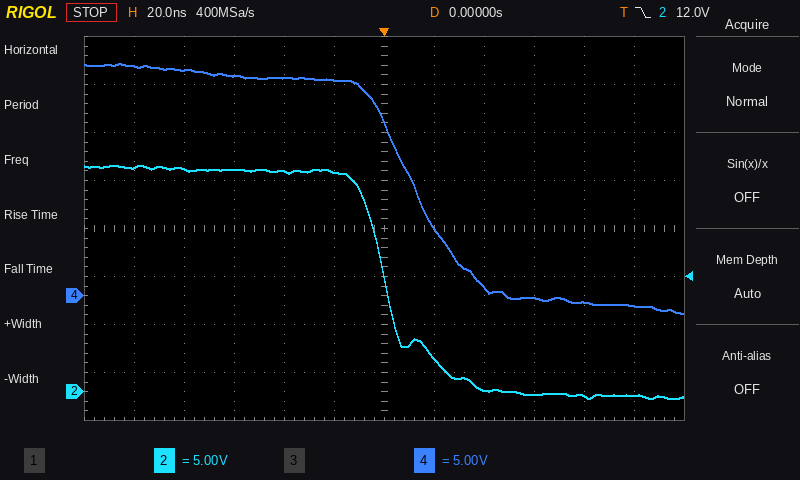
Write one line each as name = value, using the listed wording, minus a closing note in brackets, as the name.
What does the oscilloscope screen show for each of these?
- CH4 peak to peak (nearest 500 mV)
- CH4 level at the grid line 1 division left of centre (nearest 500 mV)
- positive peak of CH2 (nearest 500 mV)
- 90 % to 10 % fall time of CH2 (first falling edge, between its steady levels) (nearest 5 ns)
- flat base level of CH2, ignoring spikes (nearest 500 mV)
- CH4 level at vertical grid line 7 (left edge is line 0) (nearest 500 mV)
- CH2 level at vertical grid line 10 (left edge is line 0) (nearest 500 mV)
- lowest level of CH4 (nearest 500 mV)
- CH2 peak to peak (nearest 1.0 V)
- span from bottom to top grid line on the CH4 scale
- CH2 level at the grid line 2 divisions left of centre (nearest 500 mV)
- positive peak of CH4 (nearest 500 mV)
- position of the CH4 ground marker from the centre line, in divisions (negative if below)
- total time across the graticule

CH4 peak to peak = 26.0 V
CH4 level at the grid line 1 division left of centre = 22.5 V
positive peak of CH2 = 23.5 V
90 % to 10 % fall time of CH2 (first falling edge, between its steady levels) = 35 ns
flat base level of CH2, ignoring spikes = -500 mV
CH4 level at vertical grid line 7 (left edge is line 0) = 7.0 V
CH2 level at vertical grid line 10 (left edge is line 0) = -500 mV
lowest level of CH4 = -2.0 V
CH2 peak to peak = 24.0 V
span from bottom to top grid line on the CH4 scale = 40 V
CH2 level at the grid line 2 divisions left of centre = 23.0 V
positive peak of CH4 = 24.0 V
position of the CH4 ground marker from the centre line, in divisions = -1.4 div
total time across the graticule = 240 ns
